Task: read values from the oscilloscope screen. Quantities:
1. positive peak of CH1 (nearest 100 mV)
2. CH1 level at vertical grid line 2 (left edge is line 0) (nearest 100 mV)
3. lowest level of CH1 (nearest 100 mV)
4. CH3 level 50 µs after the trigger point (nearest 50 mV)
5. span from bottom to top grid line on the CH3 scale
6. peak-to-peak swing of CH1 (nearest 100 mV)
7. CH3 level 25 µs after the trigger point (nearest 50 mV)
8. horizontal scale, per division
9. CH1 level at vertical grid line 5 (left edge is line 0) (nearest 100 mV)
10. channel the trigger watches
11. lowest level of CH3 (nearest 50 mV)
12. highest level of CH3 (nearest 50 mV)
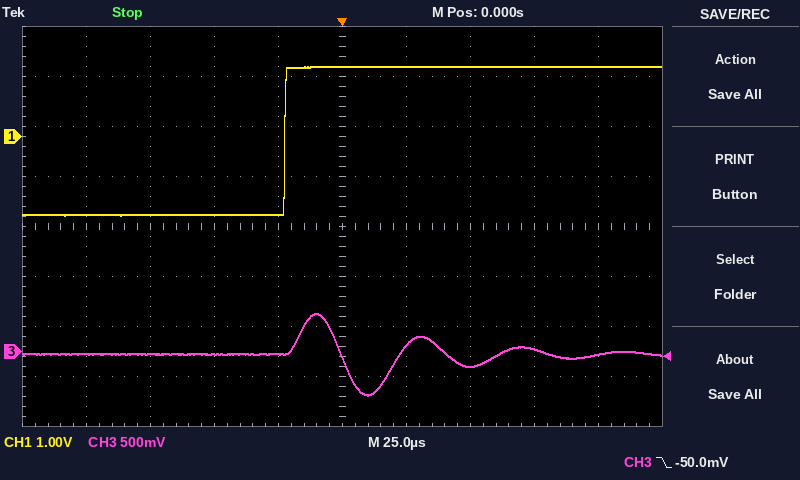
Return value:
1.4 V
-1.6 V
-1.6 V
-150 mV
4 V
3.0 V
50 mV
25 µs
1.4 V
CH3
-450 mV
400 mV
